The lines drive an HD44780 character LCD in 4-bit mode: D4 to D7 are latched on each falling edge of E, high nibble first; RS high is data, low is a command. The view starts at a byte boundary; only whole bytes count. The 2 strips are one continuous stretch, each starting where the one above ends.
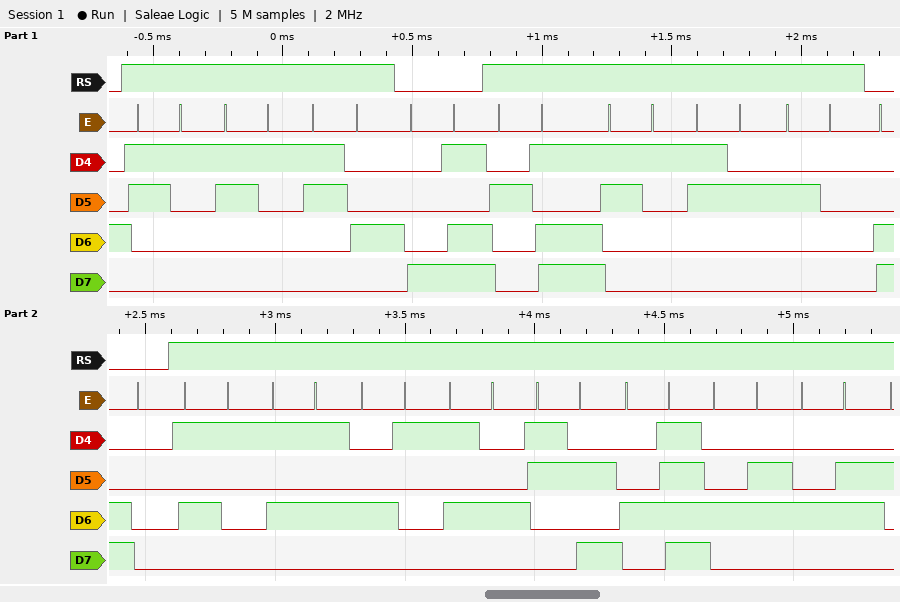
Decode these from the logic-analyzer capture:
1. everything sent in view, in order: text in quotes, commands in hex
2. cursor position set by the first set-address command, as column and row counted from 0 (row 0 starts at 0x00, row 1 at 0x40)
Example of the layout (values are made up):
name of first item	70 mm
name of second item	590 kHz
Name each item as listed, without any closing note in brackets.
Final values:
everything sent in view, in order: text in quotes, commands in hex	"114" 0x8D "-12 " 0xC0 "QUAT:OFF"
cursor position set by the first set-address command, as column and row counted from 0	column 13, row 0
